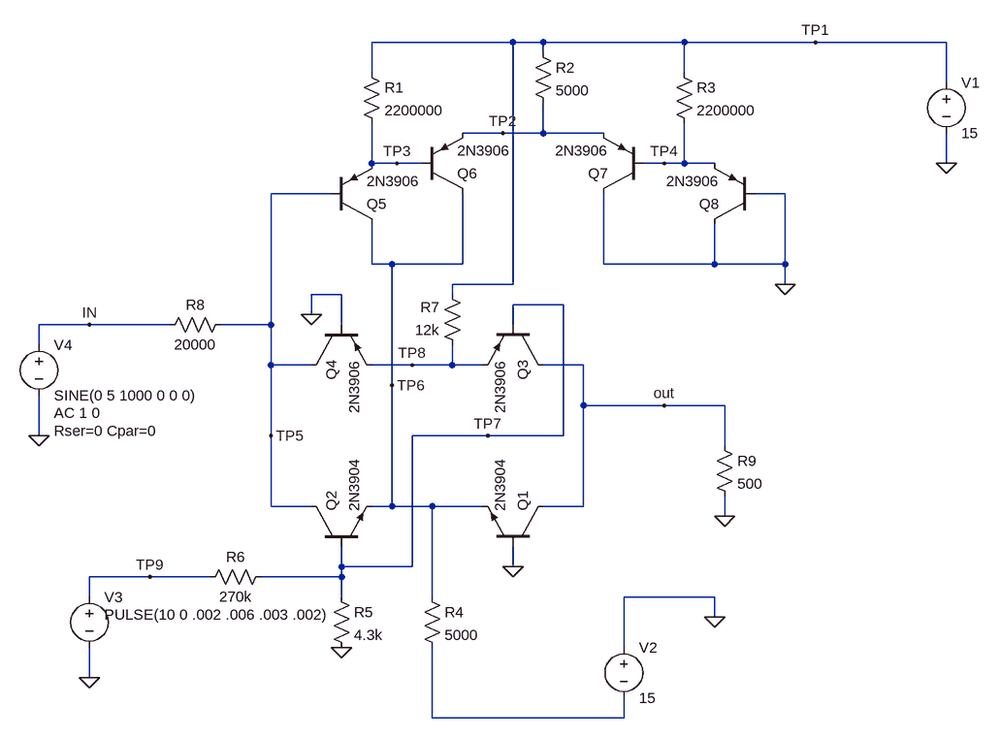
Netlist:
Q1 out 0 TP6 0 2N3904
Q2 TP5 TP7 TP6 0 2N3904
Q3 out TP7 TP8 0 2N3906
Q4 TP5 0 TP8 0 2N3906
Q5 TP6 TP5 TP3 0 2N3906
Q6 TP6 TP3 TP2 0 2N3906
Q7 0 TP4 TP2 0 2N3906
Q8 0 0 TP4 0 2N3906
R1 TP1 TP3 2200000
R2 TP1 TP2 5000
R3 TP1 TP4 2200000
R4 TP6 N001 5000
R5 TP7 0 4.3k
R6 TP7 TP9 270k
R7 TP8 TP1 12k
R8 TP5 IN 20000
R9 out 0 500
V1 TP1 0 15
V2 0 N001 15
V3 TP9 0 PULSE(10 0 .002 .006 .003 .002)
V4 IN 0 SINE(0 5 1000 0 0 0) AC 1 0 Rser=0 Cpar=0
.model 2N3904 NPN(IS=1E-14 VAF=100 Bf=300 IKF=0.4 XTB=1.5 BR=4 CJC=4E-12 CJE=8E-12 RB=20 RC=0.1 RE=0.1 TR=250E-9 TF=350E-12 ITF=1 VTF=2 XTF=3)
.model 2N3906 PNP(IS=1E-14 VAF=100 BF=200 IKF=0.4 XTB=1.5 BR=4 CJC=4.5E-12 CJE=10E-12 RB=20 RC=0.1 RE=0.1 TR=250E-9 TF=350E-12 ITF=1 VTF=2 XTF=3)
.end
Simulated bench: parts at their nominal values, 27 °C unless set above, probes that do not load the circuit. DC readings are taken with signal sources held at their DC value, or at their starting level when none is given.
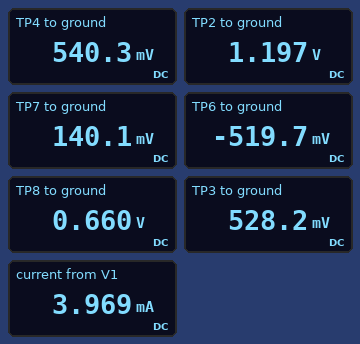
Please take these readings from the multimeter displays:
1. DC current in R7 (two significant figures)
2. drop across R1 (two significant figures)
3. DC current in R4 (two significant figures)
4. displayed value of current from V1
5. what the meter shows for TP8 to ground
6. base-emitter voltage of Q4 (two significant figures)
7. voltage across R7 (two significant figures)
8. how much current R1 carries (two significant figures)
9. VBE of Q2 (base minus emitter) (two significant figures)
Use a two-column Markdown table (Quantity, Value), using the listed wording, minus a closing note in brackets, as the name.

| Quantity | Value |
|---|---|
| DC current in R7 | 1.2 mA |
| drop across R1 | 14 V |
| DC current in R4 | 2.9 mA |
| displayed value of current from V1 | 3.969 mA |
| what the meter shows for TP8 to ground | 0.660 V |
| base-emitter voltage of Q4 | -660 mV |
| voltage across R7 | 14 V |
| how much current R1 carries | 6.6 µA |
| VBE of Q2 (base minus emitter) | 660 mV |
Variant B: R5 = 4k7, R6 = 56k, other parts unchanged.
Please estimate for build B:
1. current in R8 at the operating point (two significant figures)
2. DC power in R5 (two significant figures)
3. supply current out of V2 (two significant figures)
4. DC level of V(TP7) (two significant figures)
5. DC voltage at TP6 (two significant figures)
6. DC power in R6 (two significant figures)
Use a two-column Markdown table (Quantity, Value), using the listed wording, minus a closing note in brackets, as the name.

| Quantity | Value |
|---|---|
| current in R8 at the operating point | 1.1 µA |
| DC power in R5 | 73 µW |
| supply current out of V2 | 3.0 mA |
| DC level of V(TP7) | 590 mV |
| DC voltage at TP6 | -78 mV |
| DC power in R6 | 1.6 mW |
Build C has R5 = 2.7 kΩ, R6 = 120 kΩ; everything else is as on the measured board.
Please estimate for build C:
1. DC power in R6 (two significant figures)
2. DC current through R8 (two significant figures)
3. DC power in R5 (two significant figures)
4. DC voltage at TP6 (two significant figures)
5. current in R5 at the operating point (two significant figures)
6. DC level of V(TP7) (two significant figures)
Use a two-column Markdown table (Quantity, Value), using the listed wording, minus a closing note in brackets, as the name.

| Quantity | Value |
|---|---|
| DC power in R6 | 800 µW |
| DC current through R8 | 940 nA |
| DC power in R5 | 16 µW |
| DC voltage at TP6 | -450 mV |
| current in R5 at the operating point | 78 µA |
| DC level of V(TP7) | 210 mV |
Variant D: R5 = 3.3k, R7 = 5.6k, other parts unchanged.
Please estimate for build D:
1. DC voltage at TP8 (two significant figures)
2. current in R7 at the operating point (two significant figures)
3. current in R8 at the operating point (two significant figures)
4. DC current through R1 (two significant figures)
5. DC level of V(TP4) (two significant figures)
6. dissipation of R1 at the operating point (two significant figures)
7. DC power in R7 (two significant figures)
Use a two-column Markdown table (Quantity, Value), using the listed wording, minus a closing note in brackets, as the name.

| Quantity | Value |
|---|---|
| DC voltage at TP8 | 680 mV |
| current in R7 at the operating point | 2.6 mA |
| current in R8 at the operating point | 3.7 µA |
| DC current through R1 | 6.5 µA |
| DC level of V(TP4) | 550 mV |
| dissipation of R1 at the operating point | 94 µW |
| DC power in R7 | 37 mW |
